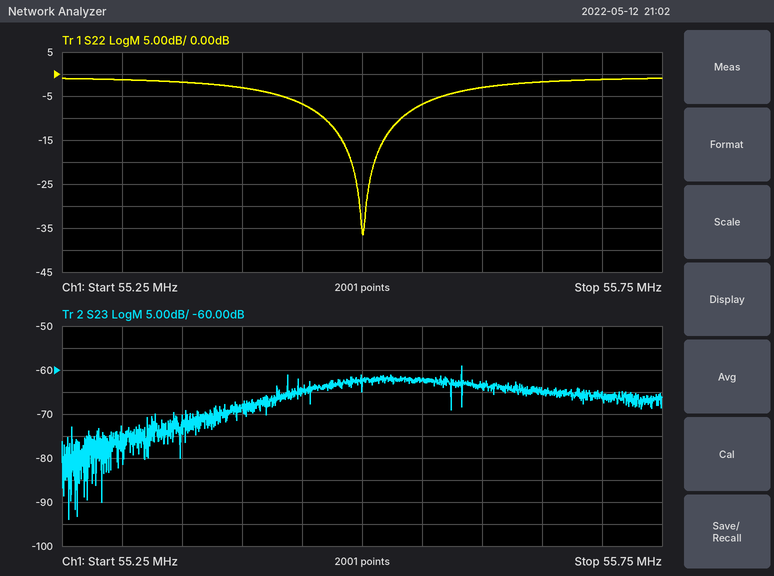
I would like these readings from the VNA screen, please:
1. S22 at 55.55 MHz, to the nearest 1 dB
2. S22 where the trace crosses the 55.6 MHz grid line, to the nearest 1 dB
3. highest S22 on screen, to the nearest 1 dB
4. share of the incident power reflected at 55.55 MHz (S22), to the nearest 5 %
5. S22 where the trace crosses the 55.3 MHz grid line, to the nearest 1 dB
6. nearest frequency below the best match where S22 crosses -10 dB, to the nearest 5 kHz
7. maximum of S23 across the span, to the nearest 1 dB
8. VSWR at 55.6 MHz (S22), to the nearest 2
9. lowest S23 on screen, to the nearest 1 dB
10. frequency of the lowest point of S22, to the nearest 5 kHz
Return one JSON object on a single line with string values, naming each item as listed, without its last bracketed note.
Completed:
{"S22 at 55.55 MHz, to the nearest 1 dB": "-7 dB", "S22 where the trace crosses the 55.6 MHz grid line, to the nearest 1 dB": "-3 dB", "highest S22 on screen, to the nearest 1 dB": "-1 dB", "share of the incident power reflected at 55.55 MHz (S22), to the nearest 5 %": "20 %", "S22 where the trace crosses the 55.3 MHz grid line, to the nearest 1 dB": "-1 dB", "nearest frequency below the best match where S22 crosses -10 dB, to the nearest 5 kHz": "55.470 MHz", "maximum of S23 across the span, to the nearest 1 dB": "-59 dB", "VSWR at 55.6 MHz (S22), to the nearest 2": "6", "lowest S23 on screen, to the nearest 1 dB": "-94 dB", "frequency of the lowest point of S22, to the nearest 5 kHz": "55.500 MHz"}
